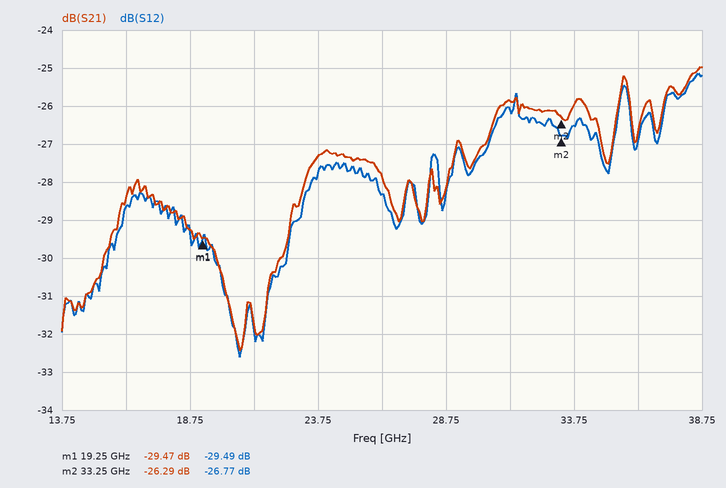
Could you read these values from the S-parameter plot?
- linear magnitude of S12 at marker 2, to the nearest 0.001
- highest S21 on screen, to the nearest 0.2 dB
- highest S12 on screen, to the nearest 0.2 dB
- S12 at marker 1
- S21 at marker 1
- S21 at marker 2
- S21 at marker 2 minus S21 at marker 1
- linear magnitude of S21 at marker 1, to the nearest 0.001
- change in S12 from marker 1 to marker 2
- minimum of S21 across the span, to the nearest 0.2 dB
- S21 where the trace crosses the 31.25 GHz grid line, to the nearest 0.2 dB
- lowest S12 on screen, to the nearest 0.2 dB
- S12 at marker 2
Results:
0.046
-25.0 dB
-25.2 dB
-29.49 dB
-29.47 dB
-26.29 dB
3.18 dB
0.034
2.72 dB
-32.4 dB
-25.8 dB
-32.6 dB
-26.77 dB
